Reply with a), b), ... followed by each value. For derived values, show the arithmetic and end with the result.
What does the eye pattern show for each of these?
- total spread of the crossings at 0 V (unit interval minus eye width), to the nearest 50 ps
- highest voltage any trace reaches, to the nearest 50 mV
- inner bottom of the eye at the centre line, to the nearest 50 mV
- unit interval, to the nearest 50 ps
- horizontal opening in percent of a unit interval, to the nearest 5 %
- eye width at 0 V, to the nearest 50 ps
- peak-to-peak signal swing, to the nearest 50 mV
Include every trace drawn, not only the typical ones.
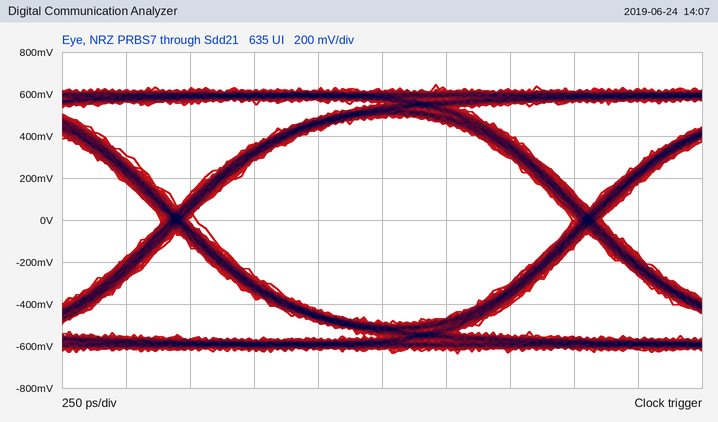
a) 150 ps
b) 650 mV
c) -500 mV
d) 1.60 ns
e) 1.45 ns / 1.60 ns ≈ 90.6 %, so 90 % to the nearest 5 %
f) 1.45 ns
g) 1.30 V
